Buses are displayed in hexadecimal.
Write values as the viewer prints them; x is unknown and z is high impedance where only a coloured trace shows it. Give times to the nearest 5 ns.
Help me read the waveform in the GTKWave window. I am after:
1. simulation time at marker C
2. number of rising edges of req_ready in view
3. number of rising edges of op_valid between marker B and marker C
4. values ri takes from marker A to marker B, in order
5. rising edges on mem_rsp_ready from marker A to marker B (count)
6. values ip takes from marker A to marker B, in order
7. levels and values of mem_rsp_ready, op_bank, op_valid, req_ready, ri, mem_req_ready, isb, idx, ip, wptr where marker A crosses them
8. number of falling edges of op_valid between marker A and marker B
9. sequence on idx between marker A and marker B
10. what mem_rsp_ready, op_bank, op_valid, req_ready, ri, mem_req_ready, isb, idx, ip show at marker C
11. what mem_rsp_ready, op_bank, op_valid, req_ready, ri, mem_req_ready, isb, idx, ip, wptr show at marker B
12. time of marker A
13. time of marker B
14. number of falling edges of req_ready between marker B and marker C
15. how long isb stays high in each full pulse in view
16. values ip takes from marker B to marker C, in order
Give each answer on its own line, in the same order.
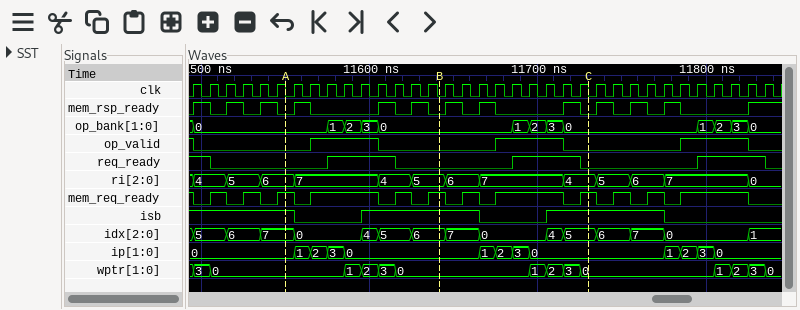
11730 ns
3
1
6, 7, 4, 5
3
0, 1, 2, 3, 0
mem_rsp_ready=0, op_bank=0, op_valid=0, req_ready=0, ri=6, mem_req_ready=1, isb=1, idx=7, ip=0, wptr=0
1
7, 0, 4, 5, 6
mem_rsp_ready=0, op_bank=0, op_valid=0, req_ready=0, ri=4, mem_req_ready=1, isb=1, idx=5, ip=0
mem_rsp_ready=0, op_bank=0, op_valid=0, req_ready=0, ri=5, mem_req_ready=1, isb=1, idx=6, ip=0, wptr=0
11550 ns
11640 ns
1
70 ns, 70 ns
0, 1, 2, 3, 0
